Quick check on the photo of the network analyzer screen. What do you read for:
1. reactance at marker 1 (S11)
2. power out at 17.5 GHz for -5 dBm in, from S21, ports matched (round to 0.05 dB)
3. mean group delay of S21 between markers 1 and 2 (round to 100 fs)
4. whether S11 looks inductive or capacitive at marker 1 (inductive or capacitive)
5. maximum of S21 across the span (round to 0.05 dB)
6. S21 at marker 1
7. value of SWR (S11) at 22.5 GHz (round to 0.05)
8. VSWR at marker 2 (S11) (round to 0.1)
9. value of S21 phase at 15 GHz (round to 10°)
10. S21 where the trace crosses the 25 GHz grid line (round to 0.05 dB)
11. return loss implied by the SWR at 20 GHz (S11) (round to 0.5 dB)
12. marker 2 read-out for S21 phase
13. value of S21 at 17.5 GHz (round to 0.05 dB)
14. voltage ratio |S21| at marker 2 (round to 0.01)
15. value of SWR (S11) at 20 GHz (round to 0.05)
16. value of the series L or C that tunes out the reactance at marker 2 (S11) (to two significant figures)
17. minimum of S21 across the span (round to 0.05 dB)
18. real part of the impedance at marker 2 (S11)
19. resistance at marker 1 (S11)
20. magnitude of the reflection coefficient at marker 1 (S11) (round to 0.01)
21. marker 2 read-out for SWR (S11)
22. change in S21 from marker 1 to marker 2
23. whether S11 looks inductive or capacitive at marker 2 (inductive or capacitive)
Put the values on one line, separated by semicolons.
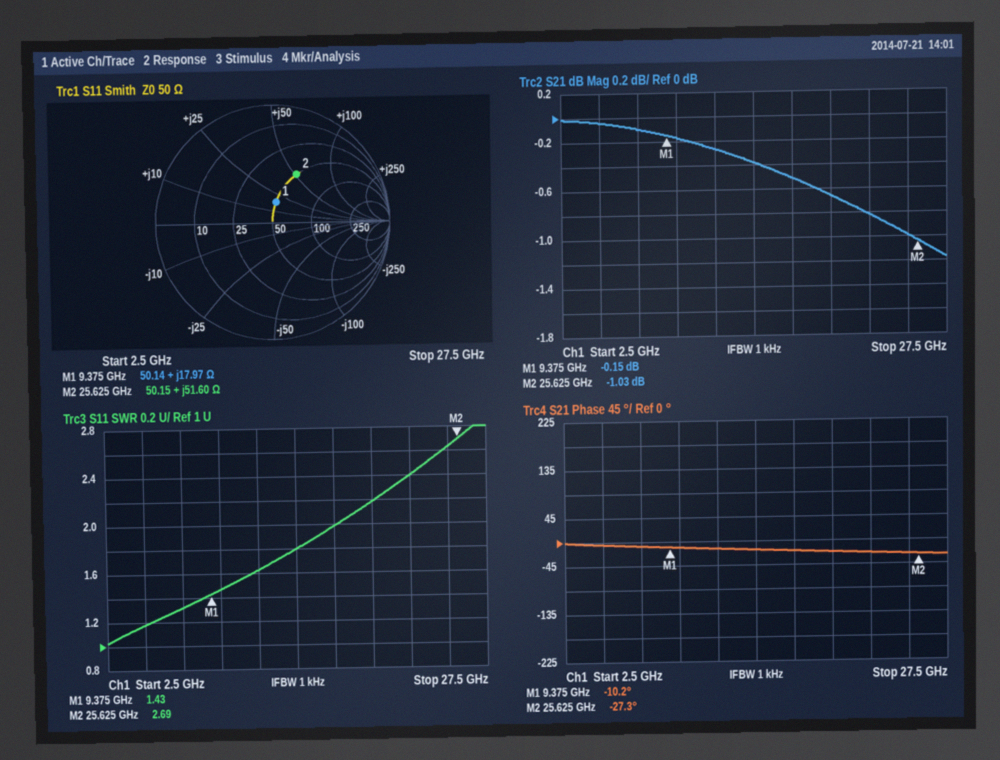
+17.97 Ω; -5.50 dBm; 2.9 ps; inductive; 0.00 dB; -0.15 dB; 2.40; 2.7; -20°; -1.00 dB; 8.5 dB; -27.3°; -0.50 dB; 0.89; 2.20; 120 fF; -1.15 dB; 50.15 Ω; 50.14 Ω; 0.18; 2.69; -0.88 dB; inductive
